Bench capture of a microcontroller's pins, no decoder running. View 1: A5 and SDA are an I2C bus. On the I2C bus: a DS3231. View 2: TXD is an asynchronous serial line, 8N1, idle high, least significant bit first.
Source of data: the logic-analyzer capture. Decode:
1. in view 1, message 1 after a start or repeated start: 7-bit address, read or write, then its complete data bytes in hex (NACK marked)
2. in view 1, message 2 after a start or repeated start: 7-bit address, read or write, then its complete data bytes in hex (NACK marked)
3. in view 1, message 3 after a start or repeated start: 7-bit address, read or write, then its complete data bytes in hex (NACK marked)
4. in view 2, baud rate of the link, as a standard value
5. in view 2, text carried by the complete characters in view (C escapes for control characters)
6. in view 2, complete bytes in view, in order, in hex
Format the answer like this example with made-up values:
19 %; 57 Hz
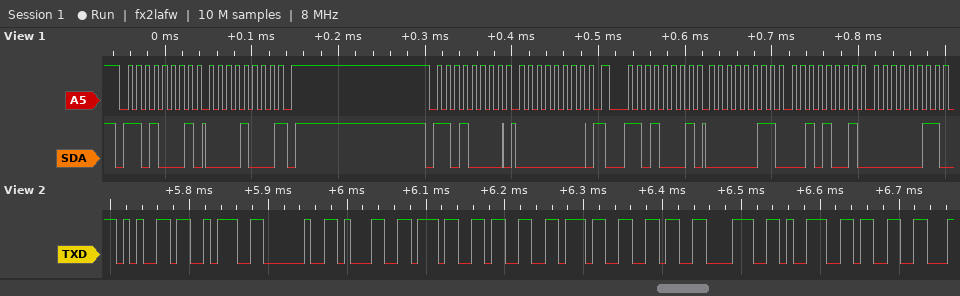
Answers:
0x68 read: 08 NACK; 0x68 write: 00; 0x68 read: 03 29 03; 115200 baud; "e: 17376893"; 0x65 0x3A 0x20 0x31 0x37 0x33 0x37 0x36 0x38 0x39 0x33
